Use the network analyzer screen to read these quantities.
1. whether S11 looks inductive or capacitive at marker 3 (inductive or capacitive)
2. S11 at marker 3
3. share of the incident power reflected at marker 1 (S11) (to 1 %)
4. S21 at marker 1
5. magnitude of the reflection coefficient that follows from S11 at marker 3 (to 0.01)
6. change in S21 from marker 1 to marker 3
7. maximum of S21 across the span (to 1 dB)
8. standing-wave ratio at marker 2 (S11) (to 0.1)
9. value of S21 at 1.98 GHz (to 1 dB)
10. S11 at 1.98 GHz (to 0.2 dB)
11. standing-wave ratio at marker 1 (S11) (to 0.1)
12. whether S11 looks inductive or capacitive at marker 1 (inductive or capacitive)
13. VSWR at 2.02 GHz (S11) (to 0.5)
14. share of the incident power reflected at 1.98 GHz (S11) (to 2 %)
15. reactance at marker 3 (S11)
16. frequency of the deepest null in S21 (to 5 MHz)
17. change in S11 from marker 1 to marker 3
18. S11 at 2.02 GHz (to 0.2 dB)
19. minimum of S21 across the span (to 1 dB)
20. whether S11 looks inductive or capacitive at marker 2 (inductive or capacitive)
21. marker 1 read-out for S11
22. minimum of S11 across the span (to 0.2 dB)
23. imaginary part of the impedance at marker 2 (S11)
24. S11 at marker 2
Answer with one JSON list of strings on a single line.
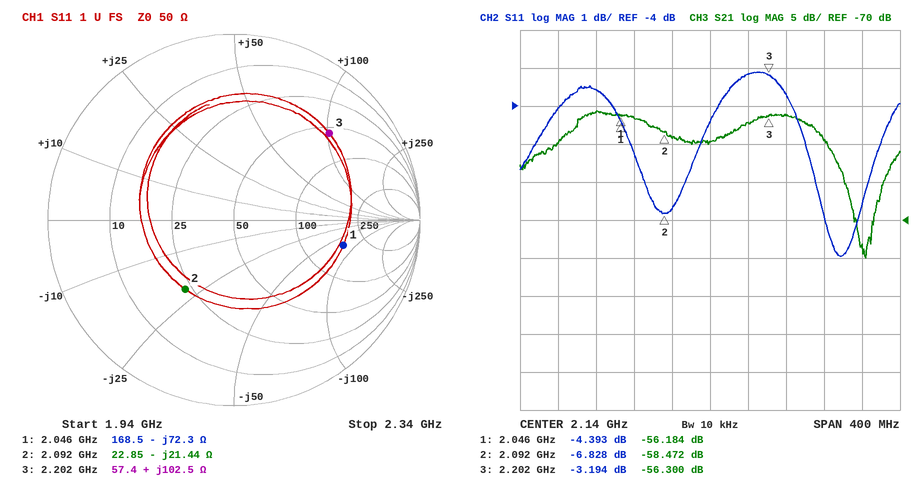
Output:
["inductive", "-3.194 dB", "36 %", "-56.184 dB", "0.69", "-0.116 dB", "-56 dB", "2.7", "-60 dB", "-4.0 dB", "4.0", "capacitive", "5.0", "40 %", "+102.5 Ω", "2.305 GHz", "1.199 dB", "-3.6 dB", "-75 dB", "capacitive", "-4.393 dB", "-8.0 dB", "-21.44 Ω", "-6.828 dB"]
